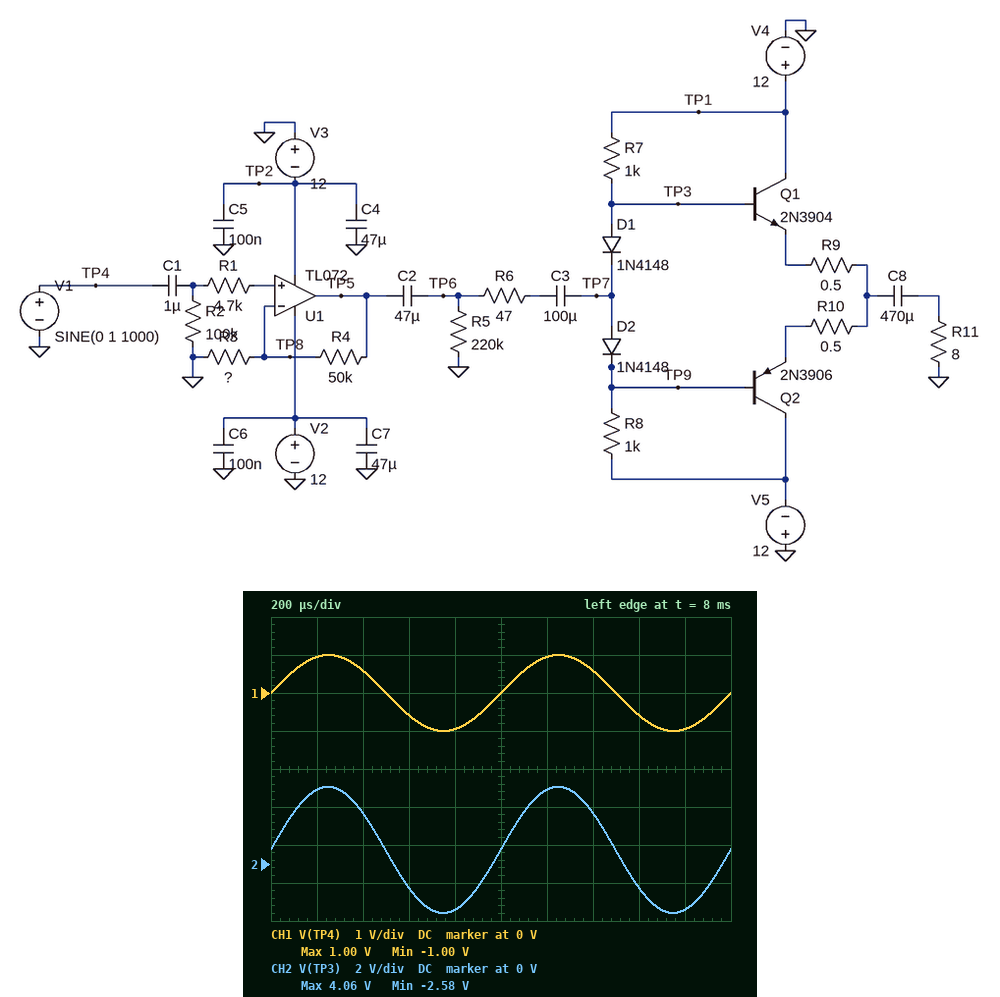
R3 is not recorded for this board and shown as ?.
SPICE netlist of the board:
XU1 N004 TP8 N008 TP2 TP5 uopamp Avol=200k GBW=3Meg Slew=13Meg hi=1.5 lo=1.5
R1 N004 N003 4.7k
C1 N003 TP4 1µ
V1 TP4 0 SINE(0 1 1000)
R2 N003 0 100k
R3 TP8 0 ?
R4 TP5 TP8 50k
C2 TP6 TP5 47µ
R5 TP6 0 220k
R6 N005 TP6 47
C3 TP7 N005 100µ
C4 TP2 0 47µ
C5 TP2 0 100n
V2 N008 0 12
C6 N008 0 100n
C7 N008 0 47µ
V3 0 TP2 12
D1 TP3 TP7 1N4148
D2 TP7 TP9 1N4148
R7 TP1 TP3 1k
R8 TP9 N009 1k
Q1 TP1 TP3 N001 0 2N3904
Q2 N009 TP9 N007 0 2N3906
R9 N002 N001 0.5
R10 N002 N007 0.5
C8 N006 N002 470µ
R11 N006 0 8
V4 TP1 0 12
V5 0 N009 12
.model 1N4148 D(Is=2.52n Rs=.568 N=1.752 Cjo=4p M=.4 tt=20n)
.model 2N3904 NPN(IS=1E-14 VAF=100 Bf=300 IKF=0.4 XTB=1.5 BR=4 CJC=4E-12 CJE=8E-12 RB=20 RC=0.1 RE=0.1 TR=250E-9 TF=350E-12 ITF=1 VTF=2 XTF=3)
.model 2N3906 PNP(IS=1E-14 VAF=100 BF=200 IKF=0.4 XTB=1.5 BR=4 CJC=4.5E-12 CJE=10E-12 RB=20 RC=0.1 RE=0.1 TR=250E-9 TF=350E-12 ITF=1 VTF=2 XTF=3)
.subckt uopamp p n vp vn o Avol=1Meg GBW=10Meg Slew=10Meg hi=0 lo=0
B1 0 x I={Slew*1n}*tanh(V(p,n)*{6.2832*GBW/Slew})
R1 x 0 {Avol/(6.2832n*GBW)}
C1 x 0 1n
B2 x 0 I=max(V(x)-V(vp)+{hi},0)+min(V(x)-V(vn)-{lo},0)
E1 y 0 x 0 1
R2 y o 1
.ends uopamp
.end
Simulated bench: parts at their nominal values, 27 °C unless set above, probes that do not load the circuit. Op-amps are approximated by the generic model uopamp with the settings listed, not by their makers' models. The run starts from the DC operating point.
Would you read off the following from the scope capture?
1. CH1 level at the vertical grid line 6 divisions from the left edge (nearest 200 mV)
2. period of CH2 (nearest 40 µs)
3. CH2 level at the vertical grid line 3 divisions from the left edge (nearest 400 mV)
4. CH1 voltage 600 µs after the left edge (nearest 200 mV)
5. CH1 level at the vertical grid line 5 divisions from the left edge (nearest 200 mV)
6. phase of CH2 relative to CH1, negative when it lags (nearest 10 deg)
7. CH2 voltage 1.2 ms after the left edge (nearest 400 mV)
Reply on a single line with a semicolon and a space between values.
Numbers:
1.0 V; 1.00 ms; -1.2 V; -600 mV; 0 V; 0 deg; 4.0 V
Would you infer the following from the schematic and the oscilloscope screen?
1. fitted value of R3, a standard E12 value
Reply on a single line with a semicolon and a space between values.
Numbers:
18 kΩ
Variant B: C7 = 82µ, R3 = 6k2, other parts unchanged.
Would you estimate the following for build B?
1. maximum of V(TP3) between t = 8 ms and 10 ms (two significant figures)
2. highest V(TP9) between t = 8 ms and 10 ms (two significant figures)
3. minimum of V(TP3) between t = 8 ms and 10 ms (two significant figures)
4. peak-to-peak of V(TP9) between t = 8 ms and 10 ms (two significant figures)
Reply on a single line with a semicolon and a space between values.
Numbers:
6.9 V; 7.4 V; -7.4 V; 13 V
